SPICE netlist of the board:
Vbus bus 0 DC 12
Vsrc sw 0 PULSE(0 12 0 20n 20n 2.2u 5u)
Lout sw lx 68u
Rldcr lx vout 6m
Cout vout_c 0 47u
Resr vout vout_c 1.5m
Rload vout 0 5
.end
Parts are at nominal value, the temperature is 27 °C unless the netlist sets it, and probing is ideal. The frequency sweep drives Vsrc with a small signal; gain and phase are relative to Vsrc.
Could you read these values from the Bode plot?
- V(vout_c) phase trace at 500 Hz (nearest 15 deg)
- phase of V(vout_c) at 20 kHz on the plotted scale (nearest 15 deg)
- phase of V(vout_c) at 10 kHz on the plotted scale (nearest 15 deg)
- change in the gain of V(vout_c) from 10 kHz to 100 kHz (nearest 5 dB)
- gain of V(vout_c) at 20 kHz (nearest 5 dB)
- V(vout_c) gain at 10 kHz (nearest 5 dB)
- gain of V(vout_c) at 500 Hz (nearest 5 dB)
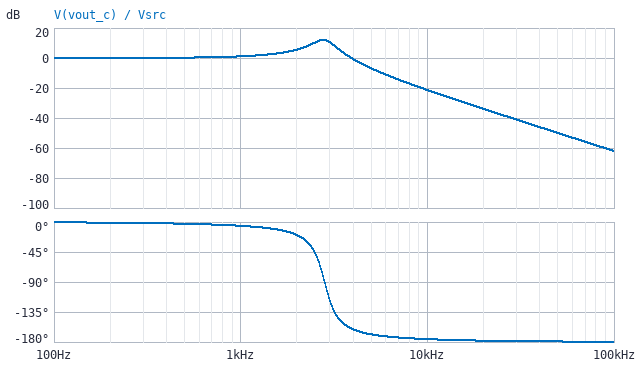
0 deg
-180 deg
-180 deg
-40 dB
-35 dB
-20 dB
0 dB
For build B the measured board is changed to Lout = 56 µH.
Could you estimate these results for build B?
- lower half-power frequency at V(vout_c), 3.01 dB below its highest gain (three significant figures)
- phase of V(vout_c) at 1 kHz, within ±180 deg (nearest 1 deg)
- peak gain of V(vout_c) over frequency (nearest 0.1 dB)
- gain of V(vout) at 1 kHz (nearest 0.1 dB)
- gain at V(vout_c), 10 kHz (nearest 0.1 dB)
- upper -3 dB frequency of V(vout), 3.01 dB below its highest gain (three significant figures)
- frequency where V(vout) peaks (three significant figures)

2.69 kHz
-5 deg
13.0 dB
0.9 dB
-19.5 dB
3.40 kHz
3.06 kHz
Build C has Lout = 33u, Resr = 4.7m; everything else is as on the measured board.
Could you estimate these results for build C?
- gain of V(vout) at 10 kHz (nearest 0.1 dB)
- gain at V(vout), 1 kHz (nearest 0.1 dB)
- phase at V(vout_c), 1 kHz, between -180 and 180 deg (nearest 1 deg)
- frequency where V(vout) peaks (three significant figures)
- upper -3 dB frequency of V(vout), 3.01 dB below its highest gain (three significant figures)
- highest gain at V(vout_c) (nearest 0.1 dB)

-14.2 dB
0.5 dB
-3 deg
4.01 kHz
4.36 kHz
14.9 dB
